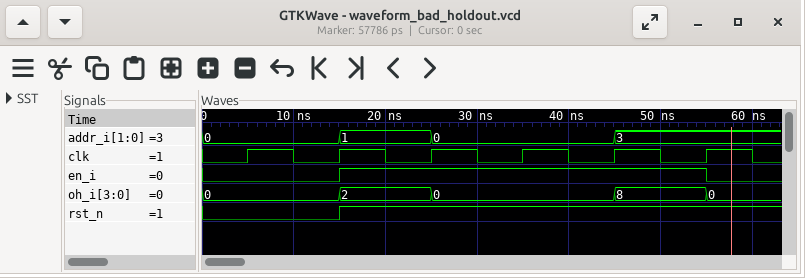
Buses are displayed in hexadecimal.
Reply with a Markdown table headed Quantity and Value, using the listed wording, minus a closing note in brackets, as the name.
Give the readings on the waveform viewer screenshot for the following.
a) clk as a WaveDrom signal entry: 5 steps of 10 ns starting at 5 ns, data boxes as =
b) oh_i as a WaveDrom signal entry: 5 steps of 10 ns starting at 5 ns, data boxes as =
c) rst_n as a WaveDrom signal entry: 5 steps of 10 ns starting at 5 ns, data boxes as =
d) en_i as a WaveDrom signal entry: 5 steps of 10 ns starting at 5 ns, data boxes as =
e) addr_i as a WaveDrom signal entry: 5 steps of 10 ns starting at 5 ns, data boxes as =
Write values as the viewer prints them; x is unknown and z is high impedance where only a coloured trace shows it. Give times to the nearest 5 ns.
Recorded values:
| Quantity | Value |
|---|---|
| clk as a WaveDrom signal entry: 5 steps of 10 ns starting at 5 ns, data boxes as = | {name: 'clk', wave: 'p....'} |
| oh_i as a WaveDrom signal entry: 5 steps of 10 ns starting at 5 ns, data boxes as = | {name: 'oh_i', wave: '===.=', data: '0 2 0 8'} |
| rst_n as a WaveDrom signal entry: 5 steps of 10 ns starting at 5 ns, data boxes as = | {name: 'rst_n', wave: '01...'} |
| en_i as a WaveDrom signal entry: 5 steps of 10 ns starting at 5 ns, data boxes as = | {name: 'en_i', wave: '01...'} |
| addr_i as a WaveDrom signal entry: 5 steps of 10 ns starting at 5 ns, data boxes as = | {name: 'addr_i', wave: '===.=', data: '0 1 0 3'} |
